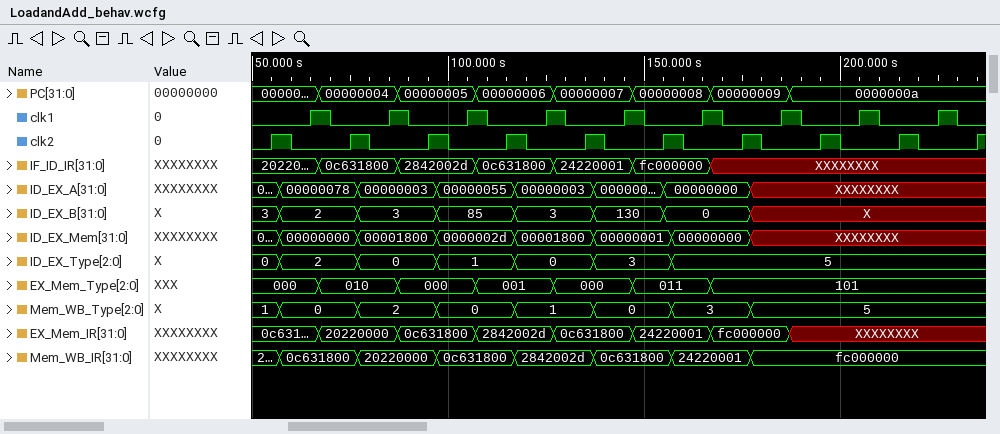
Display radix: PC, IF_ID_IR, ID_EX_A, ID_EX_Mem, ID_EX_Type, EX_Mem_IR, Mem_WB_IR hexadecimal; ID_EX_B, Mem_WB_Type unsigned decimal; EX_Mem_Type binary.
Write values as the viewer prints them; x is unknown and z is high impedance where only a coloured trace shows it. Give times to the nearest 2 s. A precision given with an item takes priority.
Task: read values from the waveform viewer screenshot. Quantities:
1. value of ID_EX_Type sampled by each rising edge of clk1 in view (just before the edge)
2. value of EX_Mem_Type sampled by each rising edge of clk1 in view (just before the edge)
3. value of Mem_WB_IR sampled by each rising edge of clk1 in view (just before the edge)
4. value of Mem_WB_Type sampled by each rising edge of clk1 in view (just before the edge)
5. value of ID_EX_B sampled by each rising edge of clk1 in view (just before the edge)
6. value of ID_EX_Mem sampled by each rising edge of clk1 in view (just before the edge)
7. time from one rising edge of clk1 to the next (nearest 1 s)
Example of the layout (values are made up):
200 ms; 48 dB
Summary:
2, 0, 1, 0, 3, 5, 5, 5, 5; 000, 010, 000, 001, 000, 011, 101, 101, 101; 0c631800, 20220000, 0c631800, 2842002d, 0c631800, 24220001, fc000000, fc000000, fc000000; 0, 2, 0, 1, 0, 3, 5, 5, 5; 2, 3, 85, 3, 130, 0, X, X, X; 00000000, 00001800, 0000002d, 00001800, 00000001, 00000000, XXXXXXXX, XXXXXXXX, XXXXXXXX; 20 s
